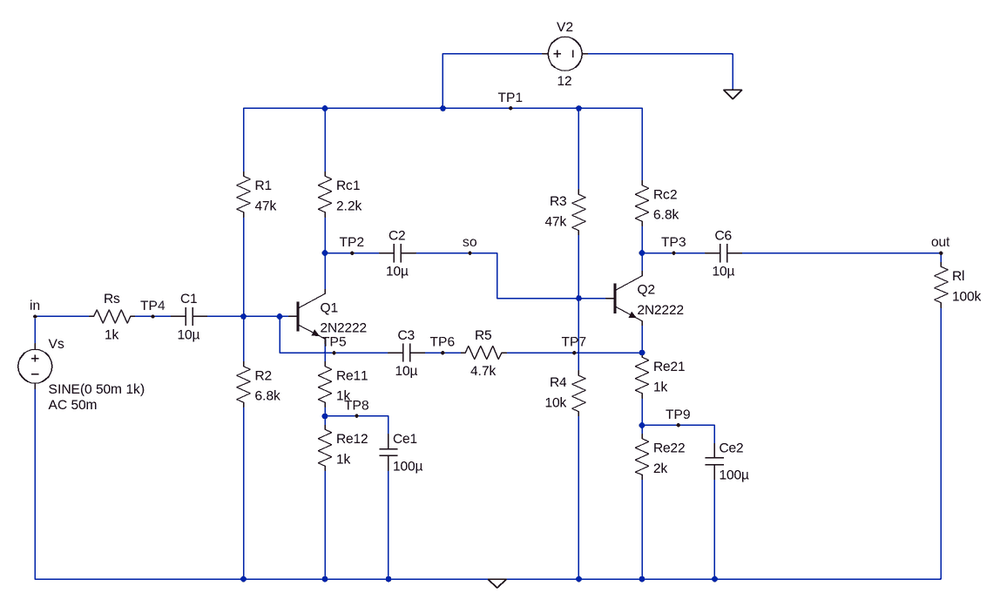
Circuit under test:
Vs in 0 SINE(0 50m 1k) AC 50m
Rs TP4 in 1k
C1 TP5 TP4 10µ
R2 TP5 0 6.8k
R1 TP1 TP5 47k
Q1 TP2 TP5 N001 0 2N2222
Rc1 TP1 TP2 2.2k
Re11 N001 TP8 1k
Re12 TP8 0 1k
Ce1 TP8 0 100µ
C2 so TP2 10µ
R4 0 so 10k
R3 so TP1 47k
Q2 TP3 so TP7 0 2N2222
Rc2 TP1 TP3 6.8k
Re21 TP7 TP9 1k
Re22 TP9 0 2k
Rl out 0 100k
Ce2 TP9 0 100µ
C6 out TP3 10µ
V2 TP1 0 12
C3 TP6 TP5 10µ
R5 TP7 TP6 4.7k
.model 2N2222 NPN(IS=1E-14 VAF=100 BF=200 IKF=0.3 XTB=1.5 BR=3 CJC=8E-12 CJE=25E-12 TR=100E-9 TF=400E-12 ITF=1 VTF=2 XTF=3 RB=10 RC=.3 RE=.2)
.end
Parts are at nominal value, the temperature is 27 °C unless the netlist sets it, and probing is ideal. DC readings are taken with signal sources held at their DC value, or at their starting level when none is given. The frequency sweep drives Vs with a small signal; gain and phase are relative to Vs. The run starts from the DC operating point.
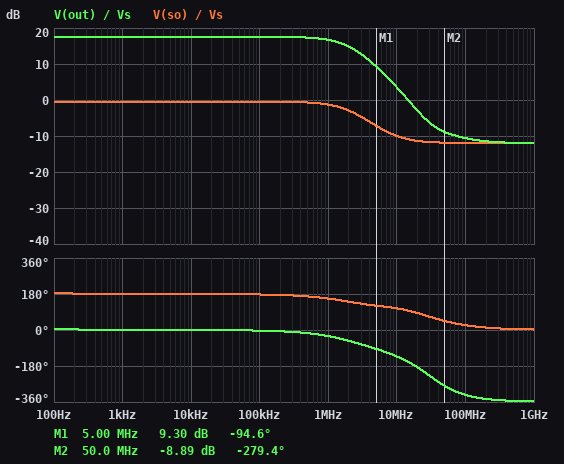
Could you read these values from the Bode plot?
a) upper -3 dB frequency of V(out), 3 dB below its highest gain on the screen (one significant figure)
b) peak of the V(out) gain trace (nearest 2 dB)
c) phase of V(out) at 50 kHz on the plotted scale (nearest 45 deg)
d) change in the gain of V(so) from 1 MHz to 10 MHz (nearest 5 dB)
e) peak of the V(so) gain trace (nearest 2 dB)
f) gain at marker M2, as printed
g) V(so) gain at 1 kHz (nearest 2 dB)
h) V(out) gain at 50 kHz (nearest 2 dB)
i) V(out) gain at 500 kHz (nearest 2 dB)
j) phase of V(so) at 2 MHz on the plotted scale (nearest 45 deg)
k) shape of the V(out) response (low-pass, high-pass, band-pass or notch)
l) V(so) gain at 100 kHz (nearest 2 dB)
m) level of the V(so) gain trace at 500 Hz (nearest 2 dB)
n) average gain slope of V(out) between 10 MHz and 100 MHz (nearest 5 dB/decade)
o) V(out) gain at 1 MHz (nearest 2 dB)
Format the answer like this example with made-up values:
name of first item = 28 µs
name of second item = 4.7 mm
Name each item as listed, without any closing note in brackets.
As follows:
upper -3 dB frequency of V(out), 3 dB below its highest gain on the screen = 2 MHz
peak of the V(out) gain trace = 18 dB
phase of V(out) at 50 kHz on the plotted scale = 0 deg
change in the gain of V(so) from 1 MHz to 10 MHz = -10 dB
peak of the V(so) gain trace = 0 dB
gain at marker M2, as printed = -8.89 dB
V(so) gain at 1 kHz = 0 dB
V(out) gain at 50 kHz = 18 dB
V(out) gain at 500 kHz = 18 dB
phase of V(so) at 2 MHz on the plotted scale = 135 deg
shape of the V(out) response = low-pass
V(so) gain at 100 kHz = 0 dB
level of the V(so) gain trace at 500 Hz = 0 dB
average gain slope of V(out) between 10 MHz and 100 MHz = -15 dB/decade
V(out) gain at 1 MHz = 16 dB
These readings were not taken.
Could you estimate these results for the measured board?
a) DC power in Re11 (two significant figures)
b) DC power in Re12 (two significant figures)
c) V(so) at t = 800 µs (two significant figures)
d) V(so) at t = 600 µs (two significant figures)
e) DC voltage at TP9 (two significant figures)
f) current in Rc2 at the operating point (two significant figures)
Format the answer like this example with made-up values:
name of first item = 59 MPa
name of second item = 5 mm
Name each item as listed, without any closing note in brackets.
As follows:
DC power in Re11 = 190 µW
DC power in Re12 = 190 µW
V(so) at t = 800 µs = 2.1 V
V(so) at t = 600 µs = 2.1 V
DC voltage at TP9 = 970 mV
current in Rc2 at the operating point = 480 µA
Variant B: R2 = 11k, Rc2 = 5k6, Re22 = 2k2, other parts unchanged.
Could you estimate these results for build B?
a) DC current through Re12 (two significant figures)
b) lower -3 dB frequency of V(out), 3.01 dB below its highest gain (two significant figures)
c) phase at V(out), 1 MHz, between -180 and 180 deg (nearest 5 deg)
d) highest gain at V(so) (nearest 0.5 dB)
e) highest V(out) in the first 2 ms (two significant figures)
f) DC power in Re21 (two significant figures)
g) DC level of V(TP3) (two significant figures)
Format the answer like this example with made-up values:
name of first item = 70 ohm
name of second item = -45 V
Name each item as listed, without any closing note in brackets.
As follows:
DC current through Re12 = 800 µA
lower -3 dB frequency of V(out), 3.01 dB below its highest gain = 8.6 Hz
phase at V(out), 1 MHz, between -180 and 180 deg = -25 deg
highest gain at V(so) = 0 dB
highest V(out) in the first 2 ms = 330 mV
DC power in Re21 = 210 µW
DC level of V(TP3) = 9.5 V
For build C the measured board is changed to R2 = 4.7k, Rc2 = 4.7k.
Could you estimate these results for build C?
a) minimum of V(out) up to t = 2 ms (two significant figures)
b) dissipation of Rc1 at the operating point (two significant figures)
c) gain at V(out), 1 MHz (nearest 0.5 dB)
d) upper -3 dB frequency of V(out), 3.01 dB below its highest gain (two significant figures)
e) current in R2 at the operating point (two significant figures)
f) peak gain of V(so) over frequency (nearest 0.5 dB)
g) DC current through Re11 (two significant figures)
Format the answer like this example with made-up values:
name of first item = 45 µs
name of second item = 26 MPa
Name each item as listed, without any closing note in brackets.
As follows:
minimum of V(out) up to t = 2 ms = -250 mV
dissipation of Rc1 at the operating point = 120 µW
gain at V(out), 1 MHz = 13.5 dB
upper -3 dB frequency of V(out), 3.01 dB below its highest gain = 2.8 MHz
current in R2 at the operating point = 230 µA
peak gain of V(so) over frequency = -1.0 dB
DC current through Re11 = 240 µA
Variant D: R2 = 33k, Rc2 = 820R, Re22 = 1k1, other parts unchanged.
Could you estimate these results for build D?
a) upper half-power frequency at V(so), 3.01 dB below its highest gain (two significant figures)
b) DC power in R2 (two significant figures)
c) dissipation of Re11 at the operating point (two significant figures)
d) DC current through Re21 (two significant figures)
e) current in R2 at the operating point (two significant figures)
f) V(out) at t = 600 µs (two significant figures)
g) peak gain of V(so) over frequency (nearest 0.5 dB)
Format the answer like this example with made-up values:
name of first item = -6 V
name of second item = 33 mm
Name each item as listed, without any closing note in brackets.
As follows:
upper half-power frequency at V(so), 3.01 dB below its highest gain = 6.7 MHz
DC power in R2 = 690 µW
dissipation of Re11 at the operating point = 4.2 mW
DC current through Re21 = 680 µA
current in R2 at the operating point = 140 µA
V(out) at t = 600 µs = -33 mV
peak gain of V(so) over frequency = 0.5 dB
